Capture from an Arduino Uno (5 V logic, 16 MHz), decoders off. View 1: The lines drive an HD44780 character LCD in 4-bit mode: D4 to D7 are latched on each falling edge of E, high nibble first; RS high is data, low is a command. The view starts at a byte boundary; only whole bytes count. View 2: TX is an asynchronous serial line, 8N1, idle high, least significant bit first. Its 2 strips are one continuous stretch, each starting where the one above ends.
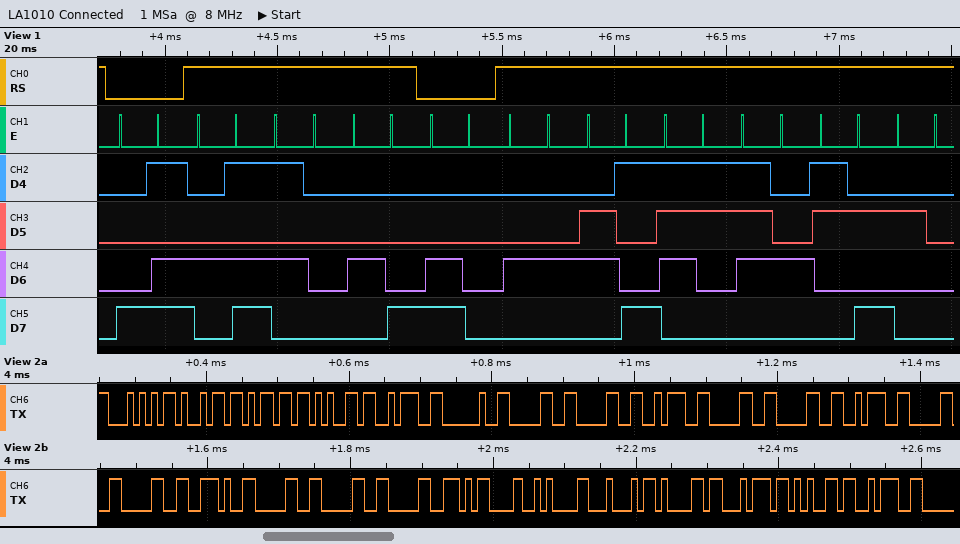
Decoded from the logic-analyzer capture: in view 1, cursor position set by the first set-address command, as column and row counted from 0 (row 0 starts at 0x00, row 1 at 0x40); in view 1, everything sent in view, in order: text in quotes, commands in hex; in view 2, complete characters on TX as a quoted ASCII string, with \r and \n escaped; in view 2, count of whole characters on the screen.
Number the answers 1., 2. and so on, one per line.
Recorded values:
1. column 13, row 0
2. 0x8D "MPH" 0xC0 "Dist: "
3. "Time: 00:00:00.000\r\nDate:"
4. 25
